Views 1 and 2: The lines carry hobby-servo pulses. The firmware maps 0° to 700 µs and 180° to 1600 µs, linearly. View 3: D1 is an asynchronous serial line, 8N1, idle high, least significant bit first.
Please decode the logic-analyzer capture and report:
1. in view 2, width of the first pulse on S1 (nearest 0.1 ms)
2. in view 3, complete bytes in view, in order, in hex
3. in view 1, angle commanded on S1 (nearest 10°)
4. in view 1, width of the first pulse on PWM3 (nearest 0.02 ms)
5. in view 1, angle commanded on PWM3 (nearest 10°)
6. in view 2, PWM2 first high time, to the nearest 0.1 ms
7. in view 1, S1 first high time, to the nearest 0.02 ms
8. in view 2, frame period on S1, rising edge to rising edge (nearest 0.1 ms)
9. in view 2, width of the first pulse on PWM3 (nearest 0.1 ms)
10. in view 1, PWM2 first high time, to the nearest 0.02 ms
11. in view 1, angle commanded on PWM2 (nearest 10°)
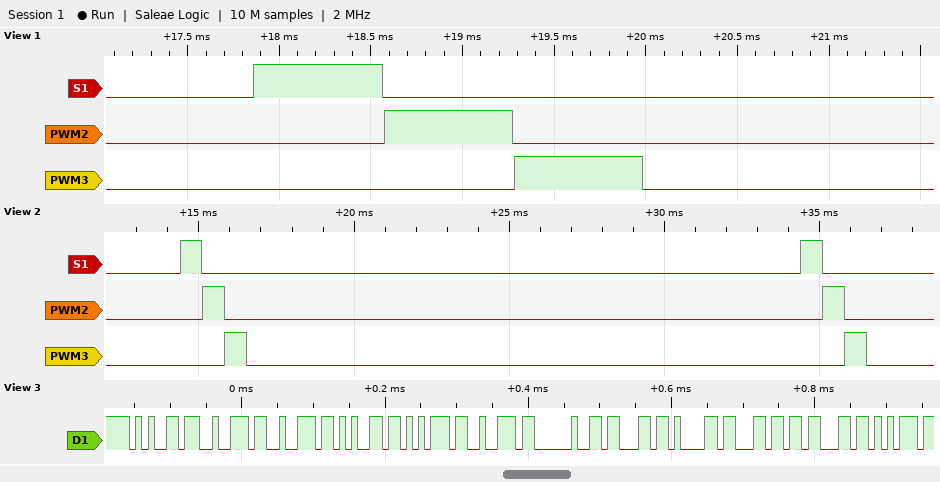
0.7 ms
65 72 72 65 75 72 20 63 61 6C 63 75
0°
0.70 ms
0°
0.7 ms
0.70 ms
20.0 ms
0.7 ms
0.70 ms
0°
